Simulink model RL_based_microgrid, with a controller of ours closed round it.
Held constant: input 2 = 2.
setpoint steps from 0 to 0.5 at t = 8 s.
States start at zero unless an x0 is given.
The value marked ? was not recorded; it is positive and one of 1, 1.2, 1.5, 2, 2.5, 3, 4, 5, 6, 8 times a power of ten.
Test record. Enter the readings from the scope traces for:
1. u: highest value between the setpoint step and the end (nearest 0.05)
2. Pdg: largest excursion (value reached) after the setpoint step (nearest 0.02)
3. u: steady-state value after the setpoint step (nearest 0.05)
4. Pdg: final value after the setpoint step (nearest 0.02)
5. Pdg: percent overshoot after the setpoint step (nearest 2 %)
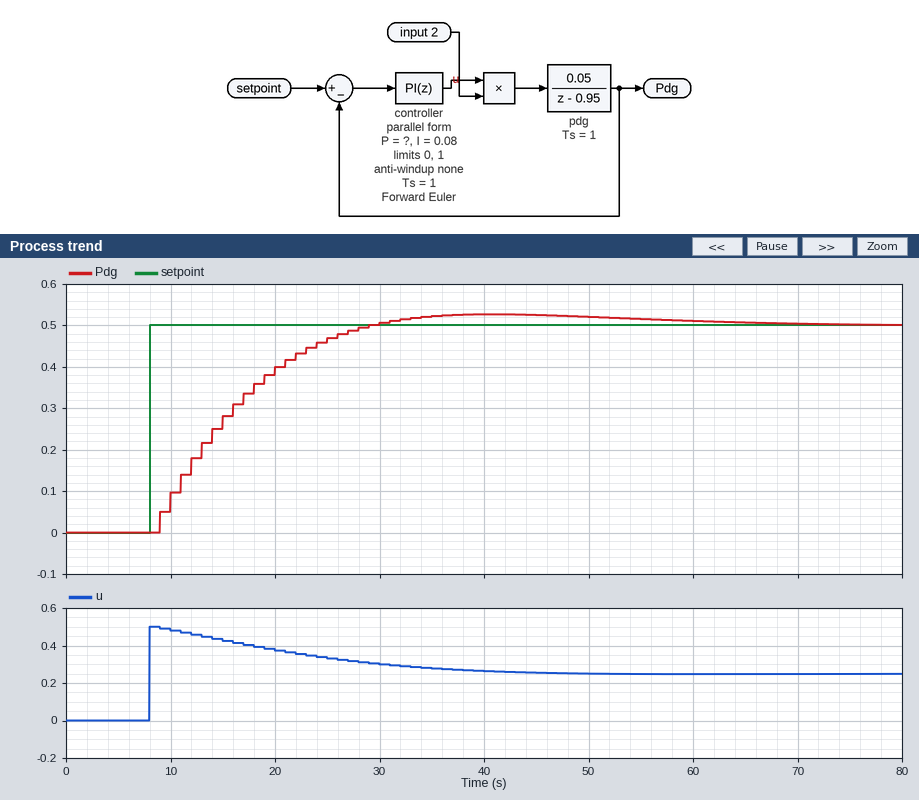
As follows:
0.50
0.52
0.25
0.50
6 %
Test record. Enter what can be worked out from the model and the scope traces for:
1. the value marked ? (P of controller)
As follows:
1
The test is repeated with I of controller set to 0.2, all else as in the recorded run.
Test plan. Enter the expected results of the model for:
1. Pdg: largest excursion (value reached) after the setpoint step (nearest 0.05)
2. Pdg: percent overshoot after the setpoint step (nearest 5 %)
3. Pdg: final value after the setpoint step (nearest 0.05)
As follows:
0.60
25 %
0.50
